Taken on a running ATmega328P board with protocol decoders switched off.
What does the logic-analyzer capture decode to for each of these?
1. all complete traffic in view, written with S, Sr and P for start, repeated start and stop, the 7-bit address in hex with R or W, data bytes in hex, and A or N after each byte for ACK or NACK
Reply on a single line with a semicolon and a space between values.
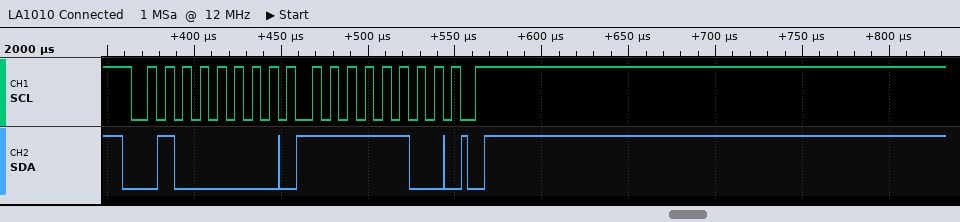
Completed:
S 20W A FC A P
